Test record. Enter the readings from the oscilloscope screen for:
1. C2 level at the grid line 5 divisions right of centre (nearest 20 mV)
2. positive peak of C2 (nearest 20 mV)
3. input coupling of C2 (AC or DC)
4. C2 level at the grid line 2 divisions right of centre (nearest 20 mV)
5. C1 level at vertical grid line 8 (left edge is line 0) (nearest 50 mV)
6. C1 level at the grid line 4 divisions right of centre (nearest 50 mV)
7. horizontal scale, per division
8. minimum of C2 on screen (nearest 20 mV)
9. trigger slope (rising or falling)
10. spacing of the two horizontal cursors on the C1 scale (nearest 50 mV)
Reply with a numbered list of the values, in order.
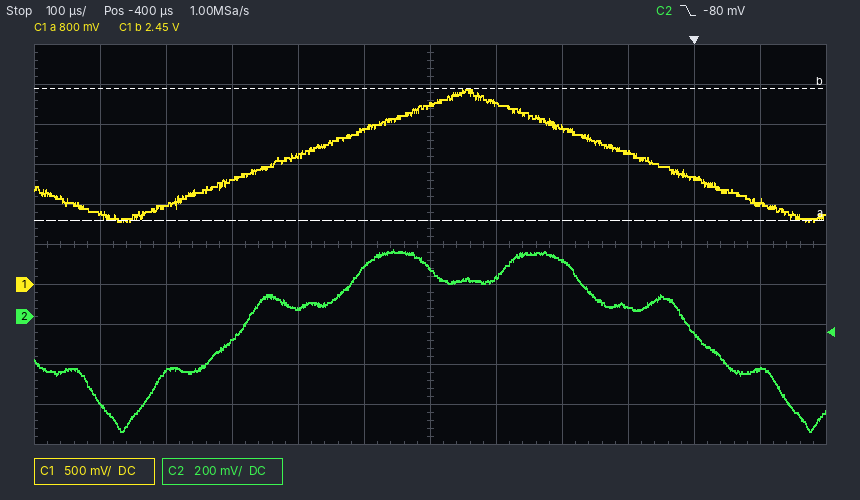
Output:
1. -260 mV
2. 340 mV
3. DC
4. 280 mV
5. 1.95 V
6. 1.35 V
7. 100 µs
8. -580 mV
9. falling
10. 1.65 V
